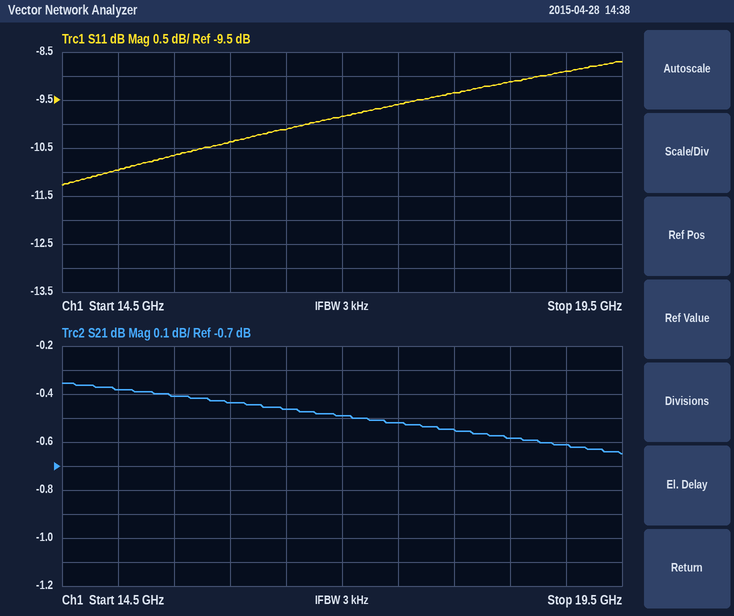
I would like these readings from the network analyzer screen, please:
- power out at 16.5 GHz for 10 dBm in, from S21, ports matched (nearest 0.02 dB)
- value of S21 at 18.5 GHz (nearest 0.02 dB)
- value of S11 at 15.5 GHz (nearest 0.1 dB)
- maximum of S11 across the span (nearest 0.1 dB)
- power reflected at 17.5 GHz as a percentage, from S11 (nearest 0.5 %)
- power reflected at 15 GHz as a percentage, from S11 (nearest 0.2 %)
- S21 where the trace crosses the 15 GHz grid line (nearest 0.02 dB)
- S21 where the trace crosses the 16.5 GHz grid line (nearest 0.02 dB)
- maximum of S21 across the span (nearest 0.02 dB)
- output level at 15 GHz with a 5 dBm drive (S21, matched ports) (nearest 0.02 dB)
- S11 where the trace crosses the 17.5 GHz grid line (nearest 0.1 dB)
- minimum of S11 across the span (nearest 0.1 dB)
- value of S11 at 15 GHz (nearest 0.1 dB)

9.54 dBm
-0.58 dB
-10.7 dB
-8.7 dB
11.0 %
8.0 %
-0.38 dB
-0.46 dB
-0.36 dB
4.62 dBm
-9.6 dB
-11.3 dB
-11.0 dB
